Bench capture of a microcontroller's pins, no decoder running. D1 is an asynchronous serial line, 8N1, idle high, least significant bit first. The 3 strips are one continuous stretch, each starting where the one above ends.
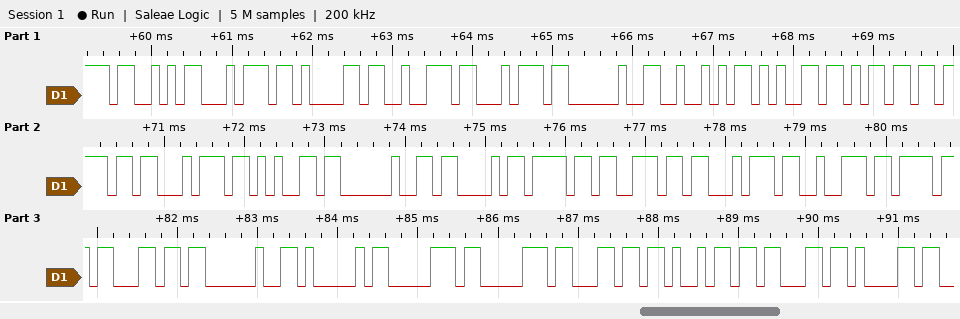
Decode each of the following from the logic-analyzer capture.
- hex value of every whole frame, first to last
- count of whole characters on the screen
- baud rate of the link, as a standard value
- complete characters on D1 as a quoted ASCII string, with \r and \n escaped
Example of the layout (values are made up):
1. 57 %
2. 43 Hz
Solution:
1. 53 74 61 72 74 20 52 65 6D 6F 74 65 20 43 6F 6E 74 72 6F 6C 20 41 70 70 6C 69 63 61
2. 28
3. 9600 baud
4. "Start Remote Control Applica"
